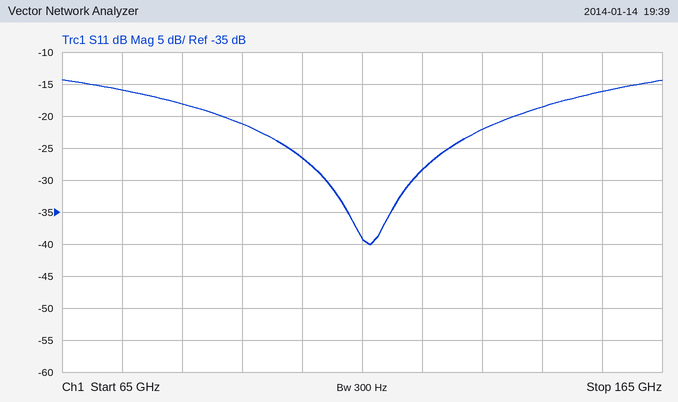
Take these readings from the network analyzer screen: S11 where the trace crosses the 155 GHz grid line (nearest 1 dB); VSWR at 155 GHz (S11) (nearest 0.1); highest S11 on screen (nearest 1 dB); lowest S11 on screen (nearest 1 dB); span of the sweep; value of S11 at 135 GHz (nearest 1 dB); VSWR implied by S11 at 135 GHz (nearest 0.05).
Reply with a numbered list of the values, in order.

1. -16 dB
2. 1.4
3. -14 dB
4. -40 dB
5. 100 GHz
6. -22 dB
7. 1.15
